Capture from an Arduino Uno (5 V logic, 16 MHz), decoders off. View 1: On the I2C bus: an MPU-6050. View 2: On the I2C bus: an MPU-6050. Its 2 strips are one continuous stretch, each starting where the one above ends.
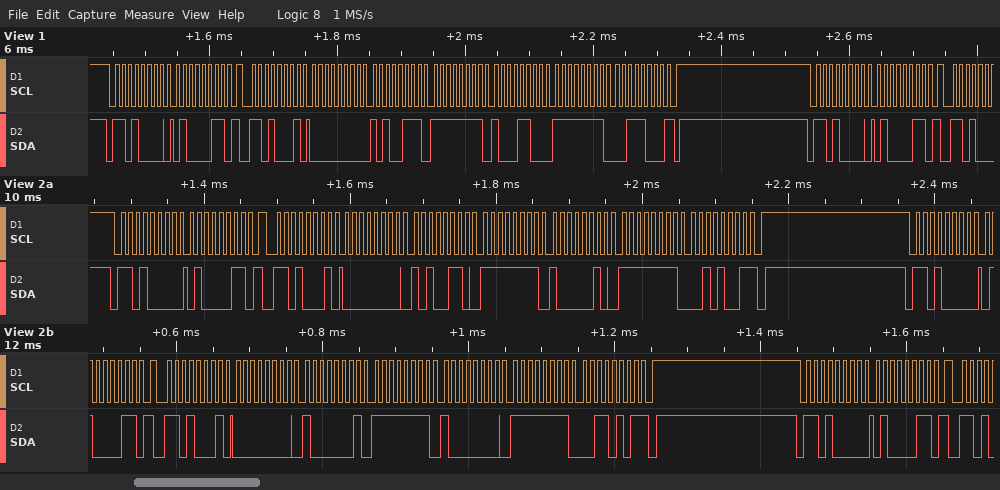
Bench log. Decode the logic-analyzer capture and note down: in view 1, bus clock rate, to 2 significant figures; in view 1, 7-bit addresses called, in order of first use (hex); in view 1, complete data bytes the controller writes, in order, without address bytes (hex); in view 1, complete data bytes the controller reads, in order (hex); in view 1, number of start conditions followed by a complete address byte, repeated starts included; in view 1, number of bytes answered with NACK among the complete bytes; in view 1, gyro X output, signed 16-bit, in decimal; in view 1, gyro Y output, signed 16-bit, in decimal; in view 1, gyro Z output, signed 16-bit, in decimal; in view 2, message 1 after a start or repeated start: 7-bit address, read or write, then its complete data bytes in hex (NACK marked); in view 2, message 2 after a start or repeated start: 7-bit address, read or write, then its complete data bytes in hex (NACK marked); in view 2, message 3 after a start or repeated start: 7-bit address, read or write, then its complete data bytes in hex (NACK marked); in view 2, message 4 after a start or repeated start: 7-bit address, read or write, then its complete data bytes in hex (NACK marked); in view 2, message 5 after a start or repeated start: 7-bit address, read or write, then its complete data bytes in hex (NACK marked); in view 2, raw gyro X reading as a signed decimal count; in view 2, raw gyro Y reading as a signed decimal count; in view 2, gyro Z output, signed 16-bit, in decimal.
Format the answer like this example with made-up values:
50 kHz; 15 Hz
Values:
100 kHz; 0x68; 43 43; 00 A7 FF 8C FF 38; 3; 1; 167; -116; -200; 0x68 write: 43; 0x68 read: 00 A6 FF 82 FF 29 NACK; 0x68 write: 43; 0x68 read: 00 81 FF 80 FF 35 NACK; 0x68 write: 43; 166; -126; -215
